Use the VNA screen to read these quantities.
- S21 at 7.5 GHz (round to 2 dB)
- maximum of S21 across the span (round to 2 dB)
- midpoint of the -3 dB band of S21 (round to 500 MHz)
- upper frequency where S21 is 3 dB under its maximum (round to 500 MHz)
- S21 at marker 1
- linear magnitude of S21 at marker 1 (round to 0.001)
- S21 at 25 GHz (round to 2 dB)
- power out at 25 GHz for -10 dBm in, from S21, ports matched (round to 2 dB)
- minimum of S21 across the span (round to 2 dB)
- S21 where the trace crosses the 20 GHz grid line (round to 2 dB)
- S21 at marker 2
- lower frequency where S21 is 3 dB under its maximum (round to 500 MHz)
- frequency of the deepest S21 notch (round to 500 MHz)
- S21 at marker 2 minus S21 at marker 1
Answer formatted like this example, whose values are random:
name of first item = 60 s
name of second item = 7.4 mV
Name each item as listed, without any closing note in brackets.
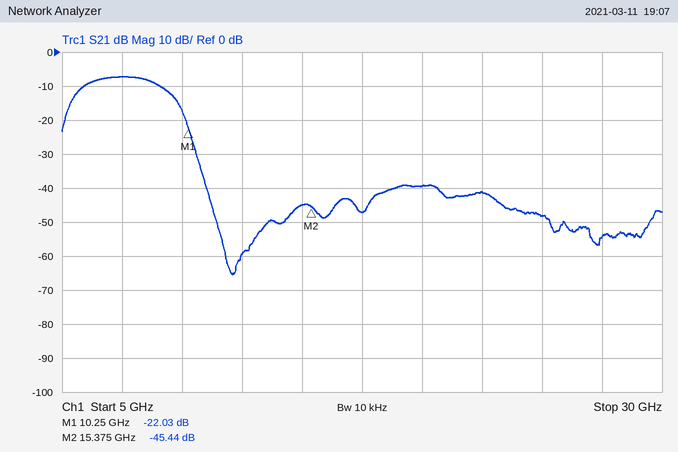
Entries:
S21 at 7.5 GHz = -8 dB
maximum of S21 across the span = -8 dB
midpoint of the -3 dB band of S21 = 7.5 GHz
upper frequency where S21 is 3 dB under its maximum = 9.0 GHz
S21 at marker 1 = -22.03 dB
linear magnitude of S21 at marker 1 = 0.079
S21 at 25 GHz = -48 dB
power out at 25 GHz for -10 dBm in, from S21, ports matched = -58 dBm
minimum of S21 across the span = -66 dB
S21 where the trace crosses the 20 GHz grid line = -40 dB
S21 at marker 2 = -45.44 dB
lower frequency where S21 is 3 dB under its maximum = 6.0 GHz
frequency of the deepest S21 notch = 12.0 GHz
S21 at marker 2 minus S21 at marker 1 = -23.41 dB
